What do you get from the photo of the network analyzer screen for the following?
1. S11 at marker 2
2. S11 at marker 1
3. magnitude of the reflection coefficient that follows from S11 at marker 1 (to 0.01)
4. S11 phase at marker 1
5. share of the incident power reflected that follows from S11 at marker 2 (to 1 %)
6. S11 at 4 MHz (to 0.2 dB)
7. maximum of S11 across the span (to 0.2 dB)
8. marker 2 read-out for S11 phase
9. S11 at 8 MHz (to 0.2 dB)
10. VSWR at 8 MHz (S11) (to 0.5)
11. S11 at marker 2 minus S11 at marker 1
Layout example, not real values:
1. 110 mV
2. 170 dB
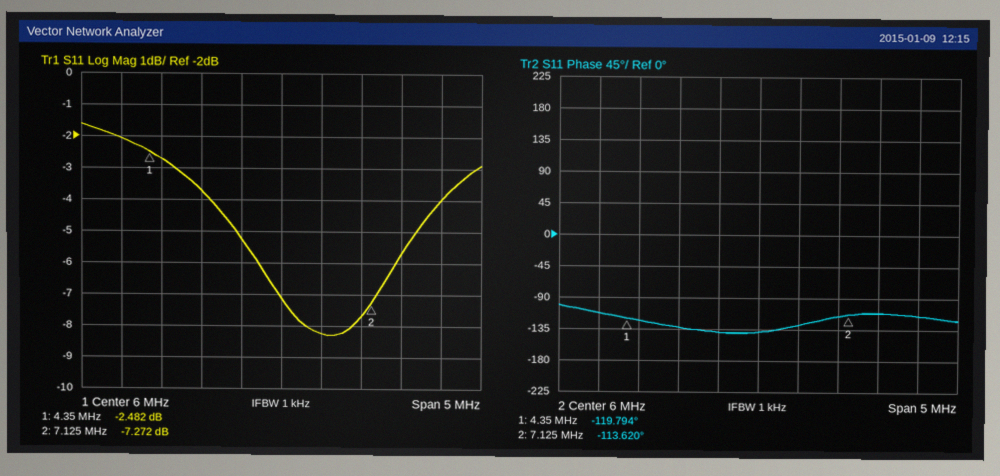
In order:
1. -7.272 dB
2. -2.482 dB
3. 0.75
4. -119.794°
5. 19 %
6. -2.0 dB
7. -1.6 dB
8. -113.620°
9. -4.0 dB
10. 4.5
11. -4.790 dB
